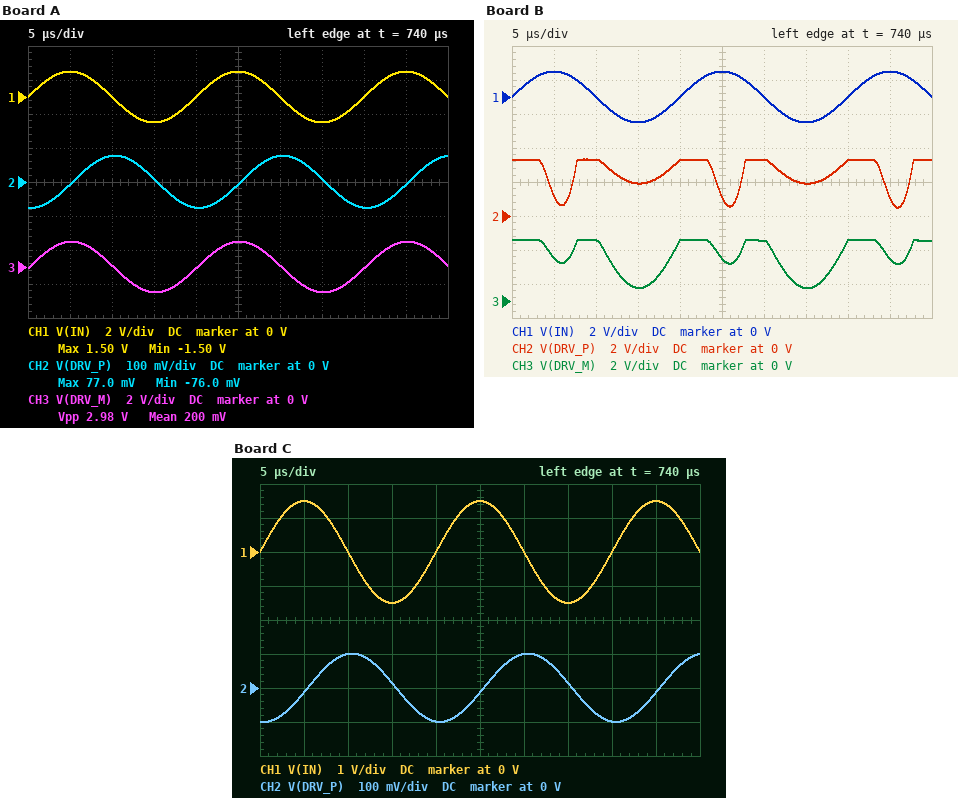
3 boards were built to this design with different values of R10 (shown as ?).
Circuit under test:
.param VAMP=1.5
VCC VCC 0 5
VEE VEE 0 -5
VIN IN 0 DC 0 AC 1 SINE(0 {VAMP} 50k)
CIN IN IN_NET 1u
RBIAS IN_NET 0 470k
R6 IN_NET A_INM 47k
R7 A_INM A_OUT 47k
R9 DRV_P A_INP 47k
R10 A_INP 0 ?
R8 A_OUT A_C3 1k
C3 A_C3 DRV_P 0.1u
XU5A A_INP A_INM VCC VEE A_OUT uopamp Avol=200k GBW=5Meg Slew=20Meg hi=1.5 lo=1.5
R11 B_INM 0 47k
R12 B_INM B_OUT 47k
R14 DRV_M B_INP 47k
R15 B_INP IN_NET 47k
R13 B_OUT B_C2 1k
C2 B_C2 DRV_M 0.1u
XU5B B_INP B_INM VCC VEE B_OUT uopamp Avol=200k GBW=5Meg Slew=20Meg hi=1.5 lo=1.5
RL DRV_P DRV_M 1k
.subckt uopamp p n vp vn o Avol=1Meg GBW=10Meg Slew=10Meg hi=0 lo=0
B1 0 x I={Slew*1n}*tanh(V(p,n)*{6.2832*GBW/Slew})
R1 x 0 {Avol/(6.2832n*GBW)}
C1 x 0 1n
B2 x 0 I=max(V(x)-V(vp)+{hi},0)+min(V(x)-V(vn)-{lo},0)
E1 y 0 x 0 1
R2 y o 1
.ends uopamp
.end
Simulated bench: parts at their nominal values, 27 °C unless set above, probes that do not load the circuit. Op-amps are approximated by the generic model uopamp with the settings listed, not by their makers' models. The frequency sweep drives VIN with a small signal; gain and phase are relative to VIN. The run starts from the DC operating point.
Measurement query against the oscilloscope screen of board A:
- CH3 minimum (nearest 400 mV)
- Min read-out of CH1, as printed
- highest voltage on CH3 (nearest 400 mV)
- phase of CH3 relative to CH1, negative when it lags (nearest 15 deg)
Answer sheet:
-1.6 V
-1.50 V
1.6 V
0 deg
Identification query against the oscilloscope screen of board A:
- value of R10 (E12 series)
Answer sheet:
22 kΩ
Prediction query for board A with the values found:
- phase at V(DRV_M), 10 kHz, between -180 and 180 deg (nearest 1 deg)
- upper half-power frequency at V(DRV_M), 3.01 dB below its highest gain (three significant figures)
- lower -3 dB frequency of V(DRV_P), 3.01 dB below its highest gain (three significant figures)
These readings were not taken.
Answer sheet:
8 deg
513 kHz
3.89 Hz
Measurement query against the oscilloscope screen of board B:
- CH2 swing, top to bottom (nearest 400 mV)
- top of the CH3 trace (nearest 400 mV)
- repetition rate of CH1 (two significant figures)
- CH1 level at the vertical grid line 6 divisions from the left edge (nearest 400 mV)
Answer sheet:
2.8 V
3.6 V
50 kHz
0 V
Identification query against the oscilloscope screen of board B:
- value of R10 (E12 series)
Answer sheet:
120 kΩ
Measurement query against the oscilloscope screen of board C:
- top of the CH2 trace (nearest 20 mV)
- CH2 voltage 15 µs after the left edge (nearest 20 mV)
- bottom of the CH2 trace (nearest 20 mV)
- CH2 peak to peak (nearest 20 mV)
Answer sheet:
100 mV
20 mV
-100 mV
200 mV
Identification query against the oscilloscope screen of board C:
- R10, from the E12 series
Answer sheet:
27 kΩ
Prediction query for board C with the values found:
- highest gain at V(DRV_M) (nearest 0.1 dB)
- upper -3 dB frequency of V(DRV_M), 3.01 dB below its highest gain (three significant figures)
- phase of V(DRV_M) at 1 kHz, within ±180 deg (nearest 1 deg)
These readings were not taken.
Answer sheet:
0 dB
425 kHz
53 deg
